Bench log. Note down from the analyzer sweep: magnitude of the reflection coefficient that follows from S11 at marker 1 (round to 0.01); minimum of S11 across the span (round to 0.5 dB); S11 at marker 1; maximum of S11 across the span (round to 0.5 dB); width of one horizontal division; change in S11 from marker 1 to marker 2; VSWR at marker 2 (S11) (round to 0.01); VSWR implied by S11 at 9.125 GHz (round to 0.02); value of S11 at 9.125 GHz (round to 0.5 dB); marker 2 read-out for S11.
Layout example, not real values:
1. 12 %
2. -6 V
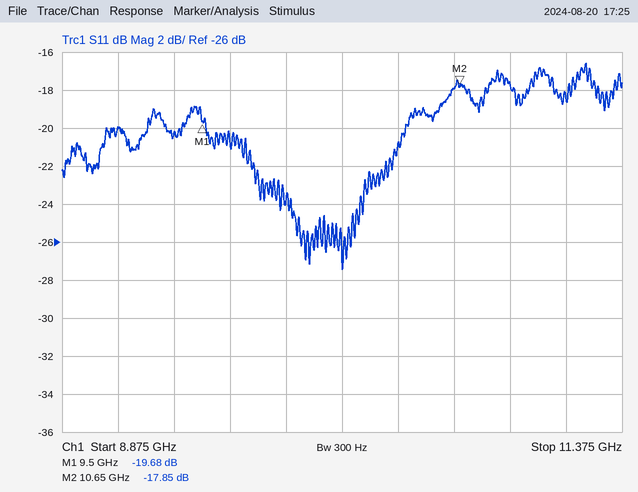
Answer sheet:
1. 0.10
2. -27.5 dB
3. -19.68 dB
4. -16.5 dB
5. 250 MHz
6. 1.83 dB
7. 1.29
8. 1.22
9. -20.0 dB
10. -17.85 dB
